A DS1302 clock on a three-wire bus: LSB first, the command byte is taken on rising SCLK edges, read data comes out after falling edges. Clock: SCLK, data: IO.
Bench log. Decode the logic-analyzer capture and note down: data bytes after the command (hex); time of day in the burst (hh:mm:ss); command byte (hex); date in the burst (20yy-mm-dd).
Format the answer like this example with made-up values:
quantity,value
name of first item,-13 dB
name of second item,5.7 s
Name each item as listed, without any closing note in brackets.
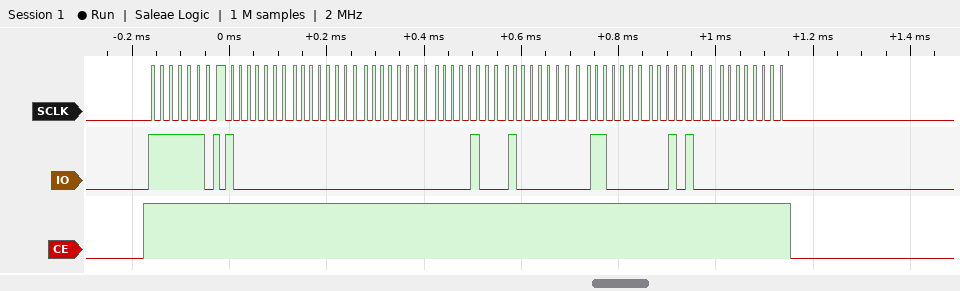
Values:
quantity,value
data bytes after the command,01 00 00 10 01 06 14 00
time of day in the burst,00:00:01
command byte,0xBF
date in the burst,2014-01-10
